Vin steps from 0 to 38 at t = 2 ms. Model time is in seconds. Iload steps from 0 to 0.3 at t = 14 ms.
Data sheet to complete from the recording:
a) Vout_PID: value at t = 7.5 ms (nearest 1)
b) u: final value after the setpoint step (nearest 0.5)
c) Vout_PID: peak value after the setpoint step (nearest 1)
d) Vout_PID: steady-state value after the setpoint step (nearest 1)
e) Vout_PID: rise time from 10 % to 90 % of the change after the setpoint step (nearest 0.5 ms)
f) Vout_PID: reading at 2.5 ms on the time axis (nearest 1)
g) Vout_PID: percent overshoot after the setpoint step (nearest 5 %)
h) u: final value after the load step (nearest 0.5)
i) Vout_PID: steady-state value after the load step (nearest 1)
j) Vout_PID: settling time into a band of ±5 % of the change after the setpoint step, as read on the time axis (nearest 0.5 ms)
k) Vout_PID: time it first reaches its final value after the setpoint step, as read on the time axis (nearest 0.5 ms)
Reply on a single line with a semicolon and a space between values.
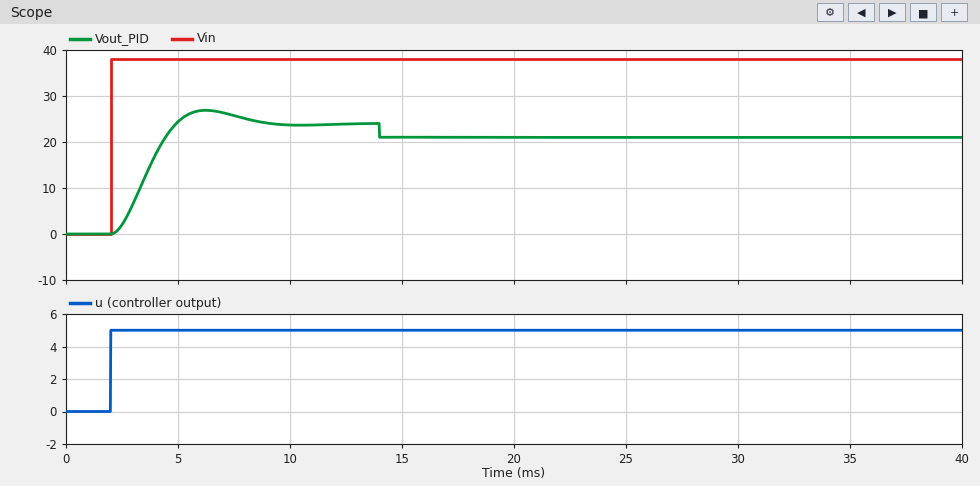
26; 5.0; 27; 24; 2.0 ms; 2; 10 %; 5.0; 21; 8.0 ms; 5.0 ms
